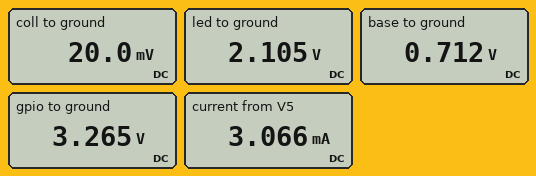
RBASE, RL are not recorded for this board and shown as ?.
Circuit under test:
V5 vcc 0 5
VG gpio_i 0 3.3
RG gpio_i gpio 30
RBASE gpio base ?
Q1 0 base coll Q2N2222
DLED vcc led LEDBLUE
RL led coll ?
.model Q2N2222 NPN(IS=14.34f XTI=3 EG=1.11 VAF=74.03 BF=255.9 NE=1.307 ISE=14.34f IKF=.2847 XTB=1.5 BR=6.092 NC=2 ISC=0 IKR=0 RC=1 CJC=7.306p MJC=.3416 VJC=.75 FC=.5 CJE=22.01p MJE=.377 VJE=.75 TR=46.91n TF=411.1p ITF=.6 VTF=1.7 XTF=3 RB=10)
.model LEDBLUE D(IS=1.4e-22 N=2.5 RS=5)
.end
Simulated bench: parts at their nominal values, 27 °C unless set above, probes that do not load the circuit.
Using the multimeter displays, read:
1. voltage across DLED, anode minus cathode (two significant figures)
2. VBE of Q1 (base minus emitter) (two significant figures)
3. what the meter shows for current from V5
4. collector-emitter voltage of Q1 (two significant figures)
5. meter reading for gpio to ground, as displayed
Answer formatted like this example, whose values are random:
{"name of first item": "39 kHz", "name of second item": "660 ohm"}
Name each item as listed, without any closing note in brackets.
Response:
{"voltage across DLED, anode minus cathode": "2.9 V", "VBE of Q1 (base minus emitter)": "690 mV", "what the meter shows for current from V5": "3.066 mA", "collector-emitter voltage of Q1": "-20 mV", "meter reading for gpio to ground, as displayed": "3.265 V"}
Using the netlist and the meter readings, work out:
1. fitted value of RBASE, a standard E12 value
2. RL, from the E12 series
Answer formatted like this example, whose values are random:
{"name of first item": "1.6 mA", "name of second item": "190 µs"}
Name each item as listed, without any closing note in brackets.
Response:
{"fitted value of RBASE, a standard E12 value": "2.2 kΩ", "RL, from the E12 series": "680 Ω"}
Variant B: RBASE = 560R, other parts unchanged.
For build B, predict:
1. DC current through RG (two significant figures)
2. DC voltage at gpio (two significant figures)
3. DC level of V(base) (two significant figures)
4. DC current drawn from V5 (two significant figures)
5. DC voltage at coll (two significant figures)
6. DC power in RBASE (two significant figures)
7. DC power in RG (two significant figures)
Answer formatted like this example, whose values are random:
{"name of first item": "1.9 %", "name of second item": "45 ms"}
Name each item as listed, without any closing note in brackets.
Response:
{"DC current through RG": "4.3 mA", "DC voltage at gpio": "3.2 V", "DC level of V(base)": "780 mV", "DC current drawn from V5": "3.1 mA", "DC voltage at coll": "11 mV", "DC power in RBASE": "10 mW", "DC power in RG": "550 µW"}
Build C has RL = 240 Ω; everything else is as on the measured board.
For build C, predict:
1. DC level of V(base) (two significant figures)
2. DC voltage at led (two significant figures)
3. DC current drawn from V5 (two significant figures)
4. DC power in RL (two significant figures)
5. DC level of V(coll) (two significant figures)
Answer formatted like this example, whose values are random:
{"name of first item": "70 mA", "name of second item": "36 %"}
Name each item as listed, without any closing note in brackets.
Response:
{"DC level of V(base)": "720 mV", "DC voltage at led": "2.0 V", "DC current drawn from V5": "7.0 mA", "DC power in RL": "12 mW", "DC level of V(coll)": "350 mV"}
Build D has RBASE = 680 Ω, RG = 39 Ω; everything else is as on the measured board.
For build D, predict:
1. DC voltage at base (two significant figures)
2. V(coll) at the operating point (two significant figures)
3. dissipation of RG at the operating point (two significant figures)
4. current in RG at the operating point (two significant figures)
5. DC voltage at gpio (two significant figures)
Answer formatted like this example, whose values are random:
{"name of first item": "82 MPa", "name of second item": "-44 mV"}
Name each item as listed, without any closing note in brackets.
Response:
{"DC voltage at base": "770 mV", "V(coll) at the operating point": "11 mV", "dissipation of RG at the operating point": "480 µW", "current in RG at the operating point": "3.5 mA", "DC voltage at gpio": "3.2 V"}
